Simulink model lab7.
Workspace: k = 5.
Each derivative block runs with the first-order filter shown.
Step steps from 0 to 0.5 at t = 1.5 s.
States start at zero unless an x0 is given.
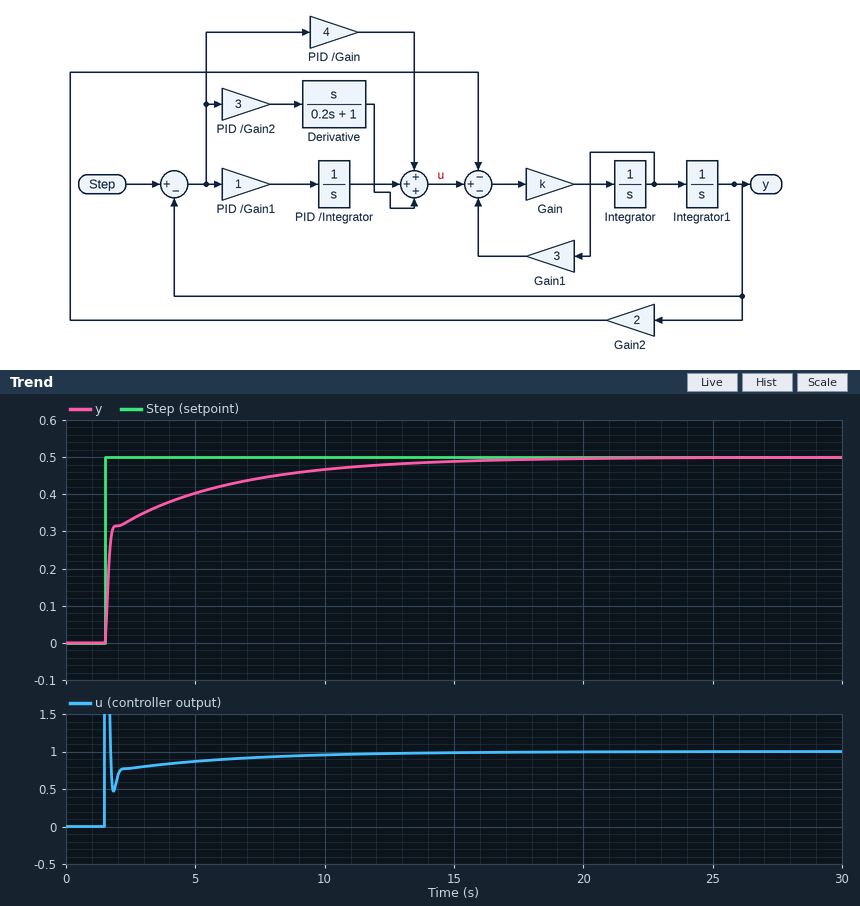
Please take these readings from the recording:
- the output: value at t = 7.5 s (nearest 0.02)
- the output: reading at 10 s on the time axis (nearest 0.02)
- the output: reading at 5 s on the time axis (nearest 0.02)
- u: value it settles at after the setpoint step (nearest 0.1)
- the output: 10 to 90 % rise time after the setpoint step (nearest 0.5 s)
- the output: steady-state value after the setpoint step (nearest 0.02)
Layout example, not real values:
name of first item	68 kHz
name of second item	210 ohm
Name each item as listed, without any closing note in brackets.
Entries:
the output: value at t = 7.5 s	0.44
the output: reading at 10 s on the time axis	0.46
the output: reading at 5 s on the time axis	0.40
u: value it settles at after the setpoint step	1.0
the output: 10 to 90 % rise time after the setpoint step	6.5 s
the output: steady-state value after the setpoint step	0.50
